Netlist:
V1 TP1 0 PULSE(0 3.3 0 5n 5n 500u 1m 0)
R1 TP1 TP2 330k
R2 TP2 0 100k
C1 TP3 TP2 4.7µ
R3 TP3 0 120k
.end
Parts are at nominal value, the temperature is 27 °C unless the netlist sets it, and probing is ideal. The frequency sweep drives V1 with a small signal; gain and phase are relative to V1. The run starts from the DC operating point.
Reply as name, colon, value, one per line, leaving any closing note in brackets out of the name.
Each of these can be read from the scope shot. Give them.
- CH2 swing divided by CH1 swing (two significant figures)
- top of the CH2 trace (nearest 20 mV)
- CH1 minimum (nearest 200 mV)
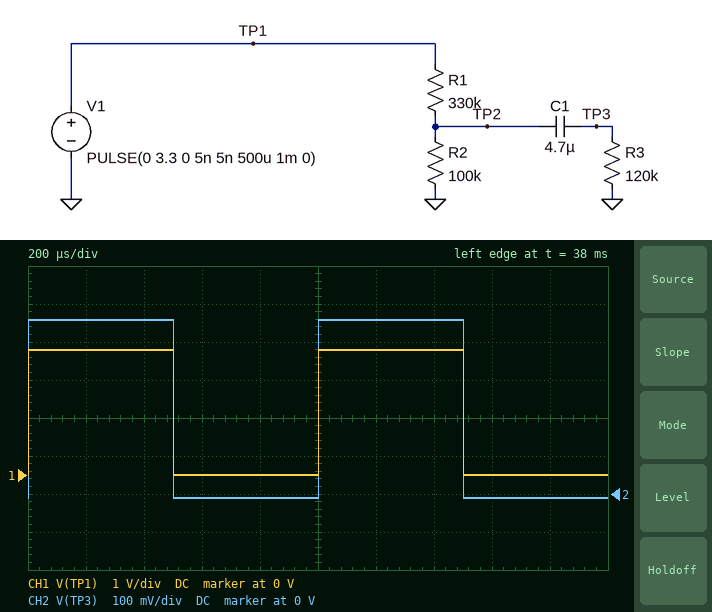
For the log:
CH2 swing divided by CH1 swing: 0.14
top of the CH2 trace: 460 mV
CH1 minimum: 0 V
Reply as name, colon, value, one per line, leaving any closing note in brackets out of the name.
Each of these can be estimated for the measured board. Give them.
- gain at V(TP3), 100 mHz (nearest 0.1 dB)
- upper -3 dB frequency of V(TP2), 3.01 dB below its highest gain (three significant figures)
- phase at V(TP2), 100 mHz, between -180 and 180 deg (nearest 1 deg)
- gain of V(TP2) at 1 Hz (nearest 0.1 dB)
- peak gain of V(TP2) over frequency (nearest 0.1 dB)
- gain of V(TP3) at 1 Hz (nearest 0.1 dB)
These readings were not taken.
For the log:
gain at V(TP3), 100 mHz: -22.9 dB
upper -3 dB frequency of V(TP2), 3.01 dB below its highest gain: 340 mHz
phase at V(TP2), 100 mHz, between -180 and 180 deg: -11 deg
gain of V(TP2) at 1 Hz: -16.8 dB
peak gain of V(TP2) over frequency: -12.7 dB
gain of V(TP3) at 1 Hz: -17.1 dB
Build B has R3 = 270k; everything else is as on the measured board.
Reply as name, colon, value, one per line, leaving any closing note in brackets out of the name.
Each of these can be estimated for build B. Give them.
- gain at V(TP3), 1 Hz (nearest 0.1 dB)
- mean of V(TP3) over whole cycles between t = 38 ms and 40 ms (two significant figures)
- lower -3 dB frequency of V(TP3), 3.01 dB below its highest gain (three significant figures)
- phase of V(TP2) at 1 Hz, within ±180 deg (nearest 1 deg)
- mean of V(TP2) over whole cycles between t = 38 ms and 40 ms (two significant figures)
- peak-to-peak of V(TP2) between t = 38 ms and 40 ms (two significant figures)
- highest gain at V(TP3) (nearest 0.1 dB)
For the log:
gain at V(TP3), 1 Hz: -14.9 dB
mean of V(TP3) over whole cycles between t = 38 ms and 40 ms: 290 mV
lower -3 dB frequency of V(TP3), 3.01 dB below its highest gain: 97.7 mHz
phase of V(TP2) at 1 Hz, within ±180 deg: -2 deg
mean of V(TP2) over whole cycles between t = 38 ms and 40 ms: 300 mV
peak-to-peak of V(TP2) between t = 38 ms and 40 ms: 600 mV
highest gain at V(TP3): -14.8 dB
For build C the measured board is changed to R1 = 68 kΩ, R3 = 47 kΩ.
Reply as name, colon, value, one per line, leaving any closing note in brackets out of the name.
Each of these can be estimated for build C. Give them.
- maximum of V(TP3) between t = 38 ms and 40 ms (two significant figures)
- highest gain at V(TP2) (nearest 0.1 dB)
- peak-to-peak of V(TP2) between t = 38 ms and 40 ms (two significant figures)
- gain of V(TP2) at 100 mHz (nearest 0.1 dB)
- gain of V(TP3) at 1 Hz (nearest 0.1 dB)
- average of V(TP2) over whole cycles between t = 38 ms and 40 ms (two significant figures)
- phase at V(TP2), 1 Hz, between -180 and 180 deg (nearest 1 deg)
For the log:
maximum of V(TP3) between t = 38 ms and 40 ms: 1.0 V
highest gain at V(TP2): -4.5 dB
peak-to-peak of V(TP2) between t = 38 ms and 40 ms: 1.1 V
gain of V(TP2) at 100 mHz: -4.7 dB
gain of V(TP3) at 1 Hz: -10.5 dB
average of V(TP2) over whole cycles between t = 38 ms and 40 ms: 570 mV
phase at V(TP2), 1 Hz, between -180 and 180 deg: -15 deg
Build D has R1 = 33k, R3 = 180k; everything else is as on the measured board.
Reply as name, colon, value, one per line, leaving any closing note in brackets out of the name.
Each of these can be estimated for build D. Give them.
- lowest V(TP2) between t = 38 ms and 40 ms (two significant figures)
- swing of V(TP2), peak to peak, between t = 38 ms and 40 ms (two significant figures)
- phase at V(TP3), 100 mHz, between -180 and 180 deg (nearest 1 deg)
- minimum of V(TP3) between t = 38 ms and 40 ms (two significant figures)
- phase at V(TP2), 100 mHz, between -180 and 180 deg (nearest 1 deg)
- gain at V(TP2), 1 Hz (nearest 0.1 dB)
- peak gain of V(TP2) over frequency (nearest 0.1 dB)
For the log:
lowest V(TP2) between t = 38 ms and 40 ms: 5.8 mV
swing of V(TP2), peak to peak, between t = 38 ms and 40 ms: 2.2 V
phase at V(TP3), 100 mHz, between -180 and 180 deg: 59 deg
minimum of V(TP3) between t = 38 ms and 40 ms: -44 mV
phase at V(TP2), 100 mHz, between -180 and 180 deg: -3 deg
gain at V(TP2), 1 Hz: -3.6 dB
peak gain of V(TP2) over frequency: -2.5 dB
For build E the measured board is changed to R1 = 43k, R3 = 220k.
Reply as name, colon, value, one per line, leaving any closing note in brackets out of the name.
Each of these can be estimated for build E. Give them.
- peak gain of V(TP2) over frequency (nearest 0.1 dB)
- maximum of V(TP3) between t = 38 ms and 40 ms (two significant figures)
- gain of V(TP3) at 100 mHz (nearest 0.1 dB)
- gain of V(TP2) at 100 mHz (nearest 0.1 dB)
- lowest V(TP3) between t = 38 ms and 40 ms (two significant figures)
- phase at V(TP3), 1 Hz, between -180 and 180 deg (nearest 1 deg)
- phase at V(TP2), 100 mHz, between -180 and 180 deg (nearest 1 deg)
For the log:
peak gain of V(TP2) over frequency: -3.1 dB
maximum of V(TP3) between t = 38 ms and 40 ms: 2.0 V
gain of V(TP3) at 100 mHz: -8.7 dB
gain of V(TP2) at 100 mHz: -3.5 dB
lowest V(TP3) between t = 38 ms and 40 ms: -34 mV
phase at V(TP3), 1 Hz, between -180 and 180 deg: 8 deg
phase at V(TP2), 100 mHz, between -180 and 180 deg: -3 deg
